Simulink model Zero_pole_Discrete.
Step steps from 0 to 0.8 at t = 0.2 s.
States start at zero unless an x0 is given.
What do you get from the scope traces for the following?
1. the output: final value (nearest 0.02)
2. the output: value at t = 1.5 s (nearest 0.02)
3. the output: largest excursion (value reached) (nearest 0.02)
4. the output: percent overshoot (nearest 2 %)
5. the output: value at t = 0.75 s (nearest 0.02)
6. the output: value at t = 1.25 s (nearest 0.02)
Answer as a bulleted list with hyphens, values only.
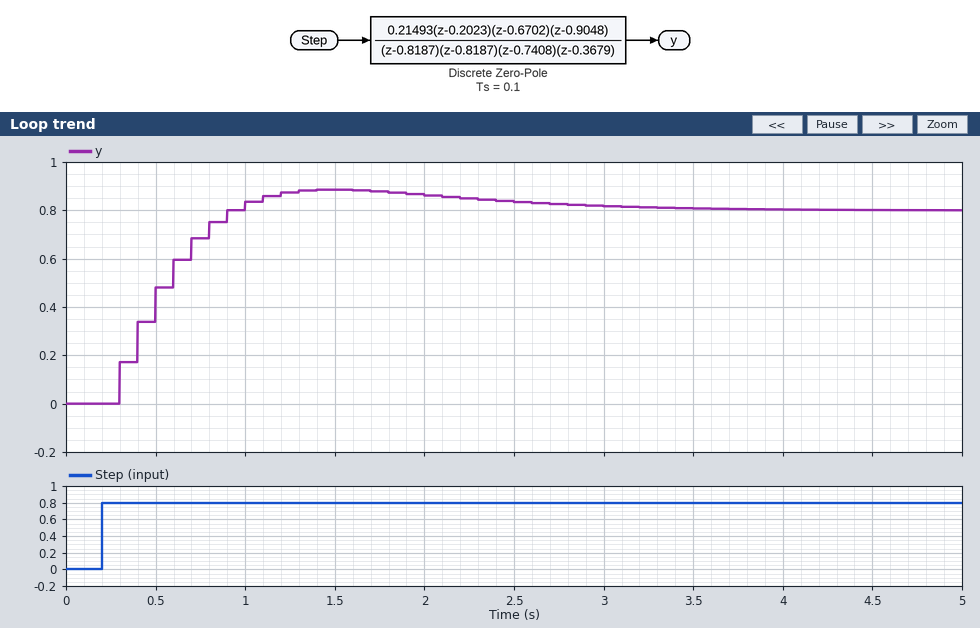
- 0.80
- 0.88
- 0.88
- 10 %
- 0.68
- 0.88
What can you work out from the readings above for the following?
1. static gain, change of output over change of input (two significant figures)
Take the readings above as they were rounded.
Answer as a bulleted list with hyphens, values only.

- 1.0
